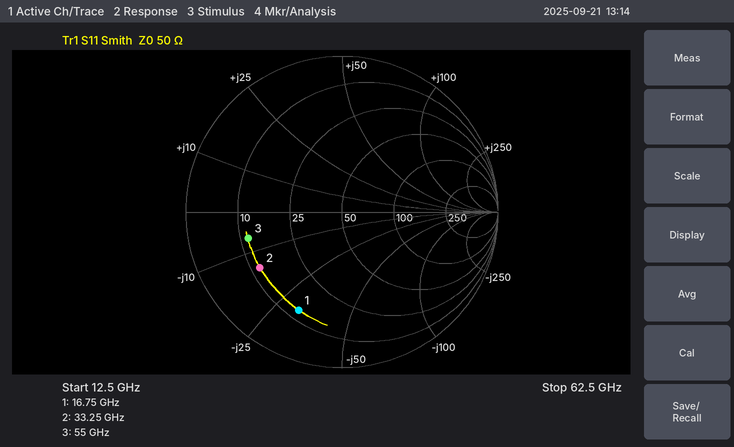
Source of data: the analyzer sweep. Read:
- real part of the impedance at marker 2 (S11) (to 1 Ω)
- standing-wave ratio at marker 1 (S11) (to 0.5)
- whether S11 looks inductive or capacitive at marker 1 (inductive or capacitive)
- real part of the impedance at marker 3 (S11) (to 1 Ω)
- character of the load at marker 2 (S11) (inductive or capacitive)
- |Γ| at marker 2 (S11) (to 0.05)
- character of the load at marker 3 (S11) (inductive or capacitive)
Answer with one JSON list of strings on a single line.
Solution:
["12 Ω", "5.5", "capacitive", "12 Ω", "capacitive", "0.65", "capacitive"]
